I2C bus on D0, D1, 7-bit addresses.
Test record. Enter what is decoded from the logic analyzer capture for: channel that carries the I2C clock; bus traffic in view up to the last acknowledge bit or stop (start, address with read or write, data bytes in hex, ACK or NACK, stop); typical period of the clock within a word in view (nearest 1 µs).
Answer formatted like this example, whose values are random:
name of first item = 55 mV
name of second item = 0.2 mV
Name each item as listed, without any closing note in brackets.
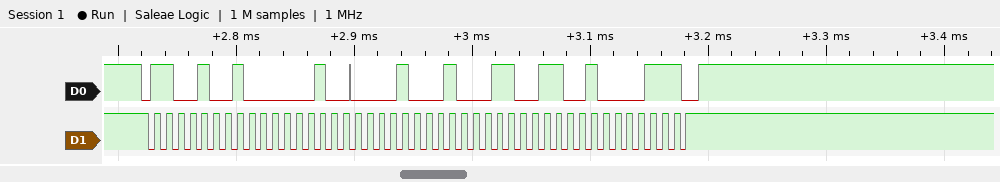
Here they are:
channel that carries the I2C clock = D1
bus traffic in view up to the last acknowledge bit or stop = start, address 64 read ACK, 04 ACK, 11 ACK, 33 ACK, 43 NACK, stop
typical period of the clock within a word in view = 10 µs
